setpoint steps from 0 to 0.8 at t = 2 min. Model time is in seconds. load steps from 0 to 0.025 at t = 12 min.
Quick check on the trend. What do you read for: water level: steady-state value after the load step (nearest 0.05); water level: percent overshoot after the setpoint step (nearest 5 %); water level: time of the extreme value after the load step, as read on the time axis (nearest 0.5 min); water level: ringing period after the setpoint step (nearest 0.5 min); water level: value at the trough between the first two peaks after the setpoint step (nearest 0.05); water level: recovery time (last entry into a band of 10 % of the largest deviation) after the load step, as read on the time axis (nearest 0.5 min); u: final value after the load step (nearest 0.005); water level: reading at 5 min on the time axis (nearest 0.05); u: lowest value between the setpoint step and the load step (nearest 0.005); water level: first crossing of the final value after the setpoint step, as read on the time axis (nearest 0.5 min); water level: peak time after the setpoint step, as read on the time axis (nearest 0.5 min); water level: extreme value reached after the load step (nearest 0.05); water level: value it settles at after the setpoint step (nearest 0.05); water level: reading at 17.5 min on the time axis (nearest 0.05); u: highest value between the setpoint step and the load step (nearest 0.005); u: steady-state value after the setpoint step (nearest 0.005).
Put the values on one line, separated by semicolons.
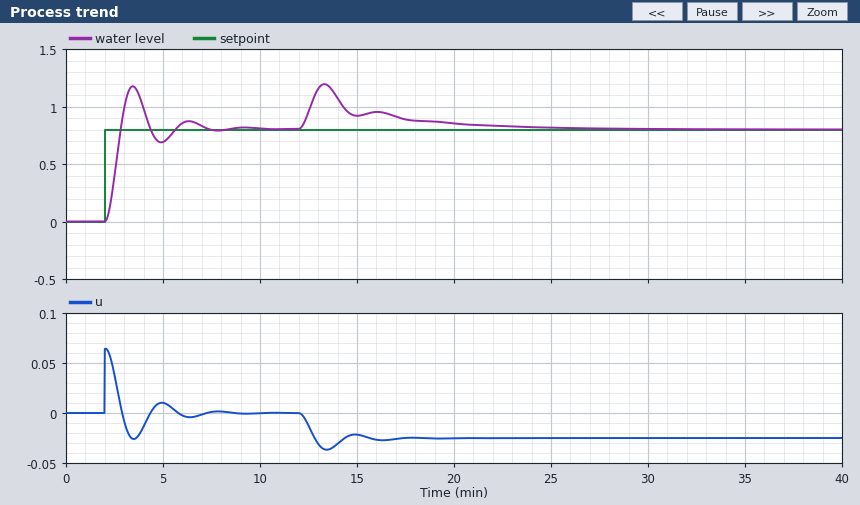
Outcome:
0.80; 45 %; 13.5 min; 3.0 min; 0.70; 21.0 min; -0.025; 0.70; -0.025; 3.0 min; 3.5 min; 1.20; 0.80; 0.90; 0.065; 0.000
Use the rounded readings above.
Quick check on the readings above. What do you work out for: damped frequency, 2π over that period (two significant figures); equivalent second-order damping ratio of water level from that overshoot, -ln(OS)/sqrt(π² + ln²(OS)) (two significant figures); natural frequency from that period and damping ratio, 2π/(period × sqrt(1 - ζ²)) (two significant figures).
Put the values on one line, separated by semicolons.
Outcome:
2.1 rad/min; 0.25; 2.2 rad/min
